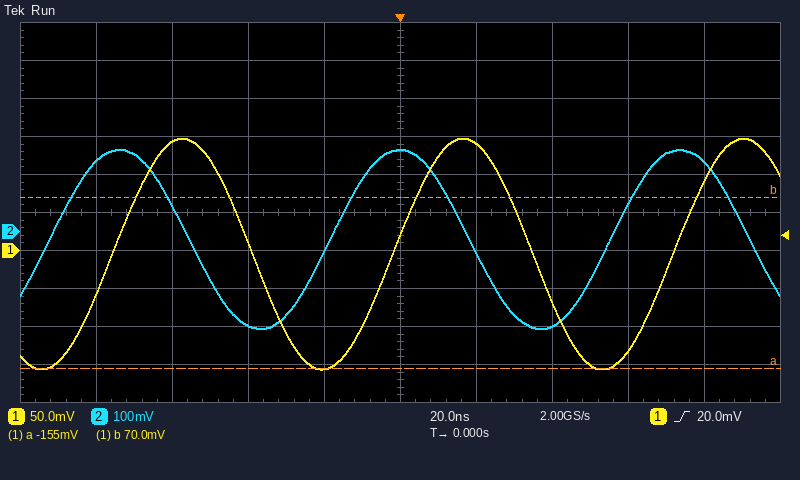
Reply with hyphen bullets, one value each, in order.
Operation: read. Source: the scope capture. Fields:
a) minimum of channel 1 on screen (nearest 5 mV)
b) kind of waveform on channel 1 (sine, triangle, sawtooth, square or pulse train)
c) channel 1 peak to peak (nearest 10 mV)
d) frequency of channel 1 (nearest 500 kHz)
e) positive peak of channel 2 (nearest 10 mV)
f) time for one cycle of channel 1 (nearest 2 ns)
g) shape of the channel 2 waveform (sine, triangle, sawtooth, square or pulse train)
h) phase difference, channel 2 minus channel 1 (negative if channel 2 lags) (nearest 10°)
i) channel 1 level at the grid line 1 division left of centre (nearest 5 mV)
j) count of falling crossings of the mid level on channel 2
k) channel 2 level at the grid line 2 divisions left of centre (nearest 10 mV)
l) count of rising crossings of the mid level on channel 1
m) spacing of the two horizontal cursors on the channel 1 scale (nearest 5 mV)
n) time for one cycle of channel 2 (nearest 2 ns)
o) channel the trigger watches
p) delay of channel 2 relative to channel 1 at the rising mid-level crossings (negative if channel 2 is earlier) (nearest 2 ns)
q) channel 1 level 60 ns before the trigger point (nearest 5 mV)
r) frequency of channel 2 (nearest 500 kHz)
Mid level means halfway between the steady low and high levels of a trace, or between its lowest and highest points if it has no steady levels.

- -155 mV
- sine
- 300 mV
- 13.5 MHz
- 220 mV
- 74 ns
- sine
- +80°
- -155 mV
- 3
- -250 mV
- 3
- 225 mV
- 74 ns
- channel 1
- -16 ns
- 145 mV
- 13.5 MHz
